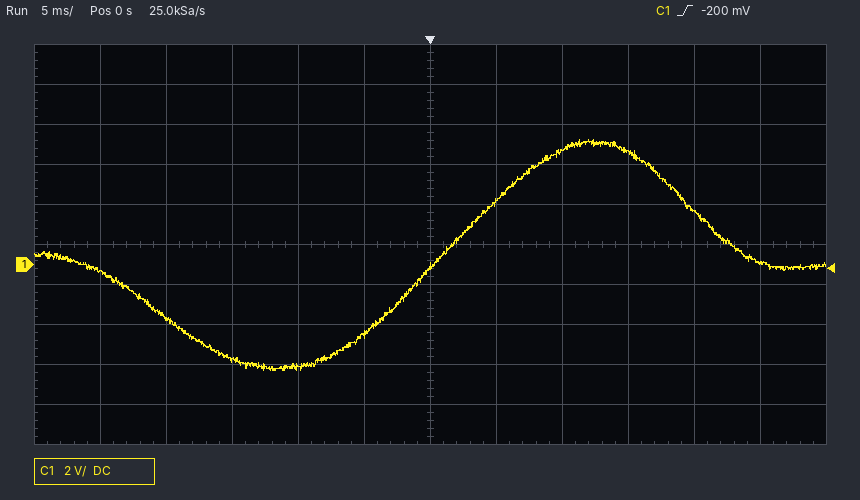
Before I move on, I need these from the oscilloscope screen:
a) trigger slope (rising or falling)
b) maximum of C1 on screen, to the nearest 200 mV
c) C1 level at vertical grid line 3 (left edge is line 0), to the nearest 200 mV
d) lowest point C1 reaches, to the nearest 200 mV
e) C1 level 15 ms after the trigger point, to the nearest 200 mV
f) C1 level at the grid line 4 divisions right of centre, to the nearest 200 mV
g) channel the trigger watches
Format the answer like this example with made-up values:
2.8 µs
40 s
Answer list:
rising
6.2 V
-4.8 V
-5.2 V
5.6 V
2.6 V
C1
